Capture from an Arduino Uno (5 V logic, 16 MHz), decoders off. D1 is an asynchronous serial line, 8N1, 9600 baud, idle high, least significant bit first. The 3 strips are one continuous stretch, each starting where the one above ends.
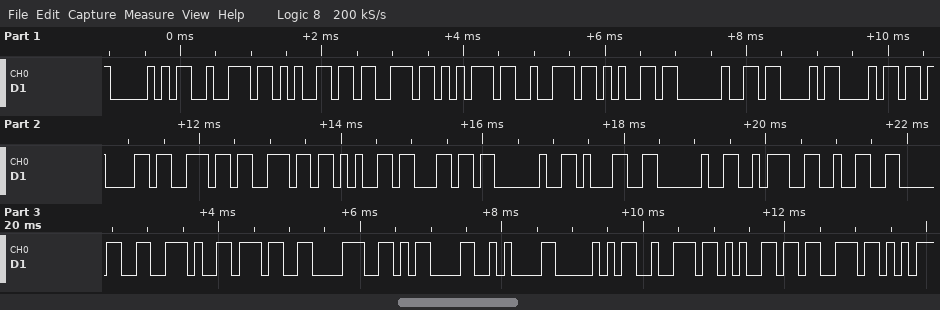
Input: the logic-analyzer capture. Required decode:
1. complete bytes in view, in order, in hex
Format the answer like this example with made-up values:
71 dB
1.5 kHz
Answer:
0x50 0x72 0x65 0x73 0x75 0x72 0x65 0x20 0x43 0x68 0x61 0x6E 0x6E 0x65 0x6C 0x20 0x31 0x20 0x3A 0x32 0x30 0x2E 0x37 0x38 0x0D 0x0A 0x50 0x72 0x65 0x73
